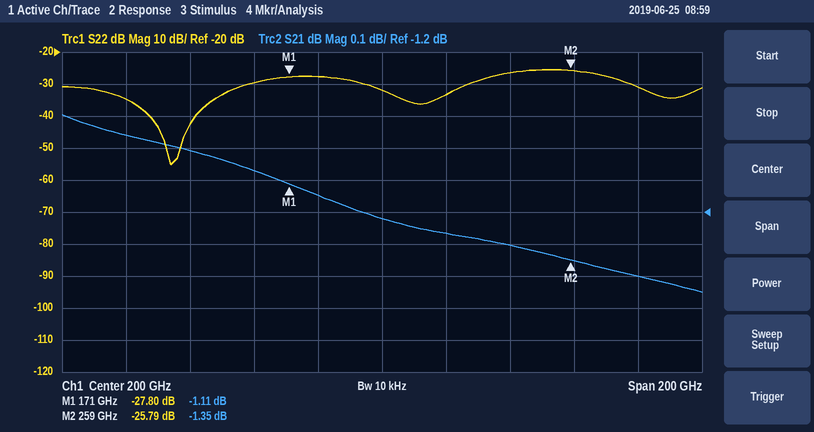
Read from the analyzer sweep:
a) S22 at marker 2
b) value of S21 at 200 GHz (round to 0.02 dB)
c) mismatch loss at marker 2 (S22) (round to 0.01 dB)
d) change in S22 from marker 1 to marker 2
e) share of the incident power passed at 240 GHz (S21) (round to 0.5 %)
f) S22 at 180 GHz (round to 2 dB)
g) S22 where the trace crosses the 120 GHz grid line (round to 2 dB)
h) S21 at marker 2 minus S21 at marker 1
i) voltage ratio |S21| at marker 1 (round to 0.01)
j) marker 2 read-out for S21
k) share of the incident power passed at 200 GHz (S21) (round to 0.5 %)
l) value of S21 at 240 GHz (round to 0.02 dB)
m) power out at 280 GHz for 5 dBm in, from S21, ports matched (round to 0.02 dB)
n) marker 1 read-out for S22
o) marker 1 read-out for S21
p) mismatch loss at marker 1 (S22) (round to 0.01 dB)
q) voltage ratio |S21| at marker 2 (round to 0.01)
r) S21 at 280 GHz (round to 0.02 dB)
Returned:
-25.79 dB
-1.22 dB
0.01 dB
2.01 dB
74.0 %
-28 dB
-34 dB
-0.24 dB
0.88
-1.35 dB
75.5 %
-1.30 dB
3.60 dBm
-27.80 dB
-1.11 dB
0.01 dB
0.86
-1.40 dB
